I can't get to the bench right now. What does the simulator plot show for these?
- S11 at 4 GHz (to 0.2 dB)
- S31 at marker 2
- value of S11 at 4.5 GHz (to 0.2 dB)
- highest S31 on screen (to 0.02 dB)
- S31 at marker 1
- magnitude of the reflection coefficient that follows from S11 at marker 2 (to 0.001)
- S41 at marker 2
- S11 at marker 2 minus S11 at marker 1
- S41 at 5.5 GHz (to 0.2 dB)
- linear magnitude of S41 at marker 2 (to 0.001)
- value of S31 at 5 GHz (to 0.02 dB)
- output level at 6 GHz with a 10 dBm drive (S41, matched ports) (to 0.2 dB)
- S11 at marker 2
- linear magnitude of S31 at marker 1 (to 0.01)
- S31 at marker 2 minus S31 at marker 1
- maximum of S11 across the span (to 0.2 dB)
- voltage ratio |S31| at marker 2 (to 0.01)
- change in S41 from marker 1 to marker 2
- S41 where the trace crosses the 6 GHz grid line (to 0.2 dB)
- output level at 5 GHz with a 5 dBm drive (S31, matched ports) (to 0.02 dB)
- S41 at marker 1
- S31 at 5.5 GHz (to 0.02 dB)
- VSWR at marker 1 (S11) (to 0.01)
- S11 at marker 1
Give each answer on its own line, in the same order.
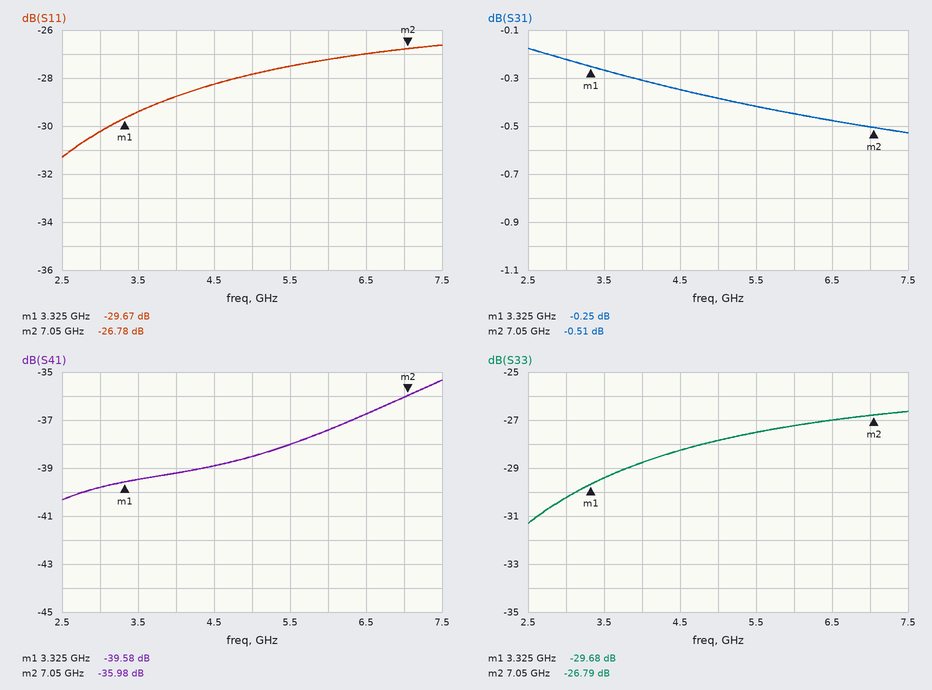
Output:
-28.8 dB
-0.51 dB
-28.2 dB
-0.18 dB
-0.25 dB
0.046
-35.98 dB
2.89 dB
-38.0 dB
0.016
-0.38 dB
-27.4 dBm
-26.78 dB
0.97
-0.26 dB
-26.6 dB
0.94
3.60 dB
-37.4 dB
4.62 dBm
-39.58 dB
-0.42 dB
1.07
-29.67 dB
